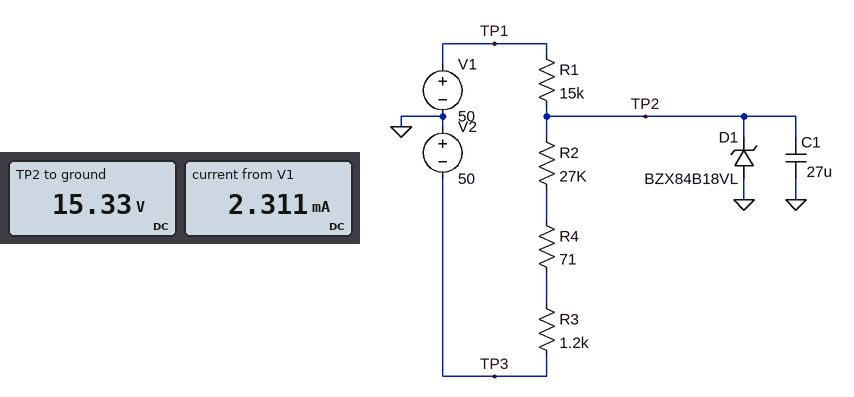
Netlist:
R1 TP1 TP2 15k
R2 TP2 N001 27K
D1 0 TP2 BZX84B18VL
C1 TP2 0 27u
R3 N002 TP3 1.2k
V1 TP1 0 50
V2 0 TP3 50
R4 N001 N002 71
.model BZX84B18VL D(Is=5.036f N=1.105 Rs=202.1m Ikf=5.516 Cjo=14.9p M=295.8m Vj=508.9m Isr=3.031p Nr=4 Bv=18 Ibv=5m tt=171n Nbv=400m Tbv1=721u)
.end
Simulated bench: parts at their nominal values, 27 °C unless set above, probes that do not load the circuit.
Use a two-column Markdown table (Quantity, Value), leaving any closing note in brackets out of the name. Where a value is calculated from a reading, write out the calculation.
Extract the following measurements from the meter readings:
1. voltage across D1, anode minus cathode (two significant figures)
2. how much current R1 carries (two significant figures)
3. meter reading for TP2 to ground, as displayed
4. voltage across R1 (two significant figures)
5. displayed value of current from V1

| Quantity | Value |
|---|---|
| voltage across D1, anode minus cathode | 0 V - 15.33 V = -15 V |
| how much current R1 carries | (50 V - 15.33 V) / 15 kΩ = 2.3 mA |
| meter reading for TP2 to ground, as displayed | 15.33 V |
| voltage across R1 | 50 V - 15.33 V = 35 V |
| displayed value of current from V1 | 2.311 mA |
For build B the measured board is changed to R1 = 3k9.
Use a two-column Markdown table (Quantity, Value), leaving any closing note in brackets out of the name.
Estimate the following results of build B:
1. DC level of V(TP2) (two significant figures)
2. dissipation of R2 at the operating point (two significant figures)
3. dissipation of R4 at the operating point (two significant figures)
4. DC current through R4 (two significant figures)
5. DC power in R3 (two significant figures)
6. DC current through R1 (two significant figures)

| Quantity | Value |
|---|---|
| DC level of V(TP2) | 18 V |
| dissipation of R2 at the operating point | 160 mW |
| dissipation of R4 at the operating point | 410 µW |
| DC current through R4 | 2.4 mA |
| DC power in R3 | 6.9 mW |
| DC current through R1 | 8.2 mA |
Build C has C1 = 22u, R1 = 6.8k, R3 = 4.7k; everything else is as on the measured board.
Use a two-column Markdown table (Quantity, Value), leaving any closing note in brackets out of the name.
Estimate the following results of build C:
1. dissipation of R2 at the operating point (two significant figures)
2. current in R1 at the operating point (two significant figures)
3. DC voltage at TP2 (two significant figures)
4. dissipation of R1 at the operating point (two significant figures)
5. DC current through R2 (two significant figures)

| Quantity | Value |
|---|---|
| dissipation of R2 at the operating point | 120 mW |
| current in R1 at the operating point | 4.7 mA |
| DC voltage at TP2 | 18 V |
| dissipation of R1 at the operating point | 150 mW |
| DC current through R2 | 2.1 mA |
